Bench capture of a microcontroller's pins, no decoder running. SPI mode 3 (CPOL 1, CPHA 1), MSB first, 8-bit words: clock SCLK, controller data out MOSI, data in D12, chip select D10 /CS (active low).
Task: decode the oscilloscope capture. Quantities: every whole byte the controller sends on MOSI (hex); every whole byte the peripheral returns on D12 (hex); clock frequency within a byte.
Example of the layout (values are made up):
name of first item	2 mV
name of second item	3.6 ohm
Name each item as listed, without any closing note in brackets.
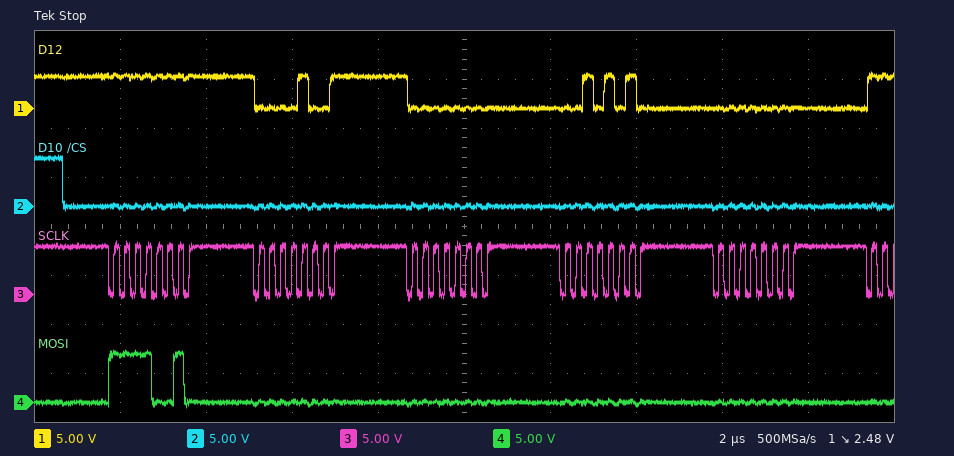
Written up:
every whole byte the controller sends on MOSI	F2 00 00 00 00
every whole byte the peripheral returns on D12	FF 09 00 2A 00
clock frequency within a byte	4 MHz
